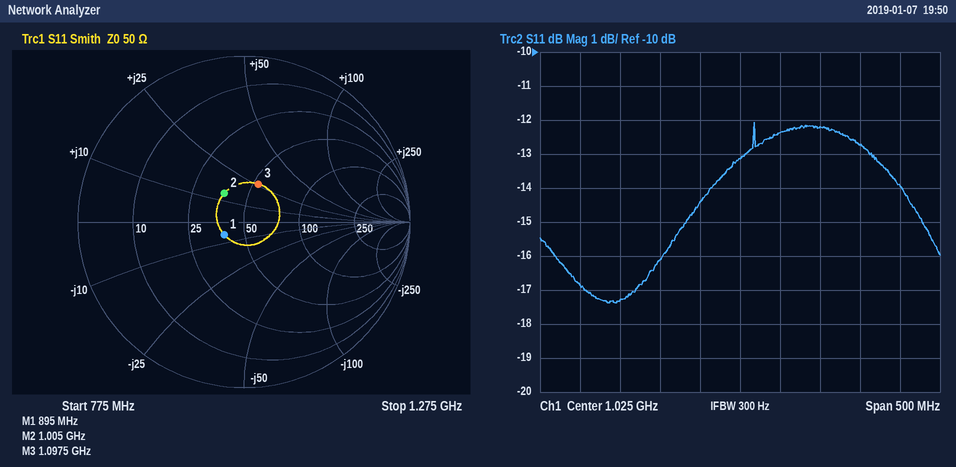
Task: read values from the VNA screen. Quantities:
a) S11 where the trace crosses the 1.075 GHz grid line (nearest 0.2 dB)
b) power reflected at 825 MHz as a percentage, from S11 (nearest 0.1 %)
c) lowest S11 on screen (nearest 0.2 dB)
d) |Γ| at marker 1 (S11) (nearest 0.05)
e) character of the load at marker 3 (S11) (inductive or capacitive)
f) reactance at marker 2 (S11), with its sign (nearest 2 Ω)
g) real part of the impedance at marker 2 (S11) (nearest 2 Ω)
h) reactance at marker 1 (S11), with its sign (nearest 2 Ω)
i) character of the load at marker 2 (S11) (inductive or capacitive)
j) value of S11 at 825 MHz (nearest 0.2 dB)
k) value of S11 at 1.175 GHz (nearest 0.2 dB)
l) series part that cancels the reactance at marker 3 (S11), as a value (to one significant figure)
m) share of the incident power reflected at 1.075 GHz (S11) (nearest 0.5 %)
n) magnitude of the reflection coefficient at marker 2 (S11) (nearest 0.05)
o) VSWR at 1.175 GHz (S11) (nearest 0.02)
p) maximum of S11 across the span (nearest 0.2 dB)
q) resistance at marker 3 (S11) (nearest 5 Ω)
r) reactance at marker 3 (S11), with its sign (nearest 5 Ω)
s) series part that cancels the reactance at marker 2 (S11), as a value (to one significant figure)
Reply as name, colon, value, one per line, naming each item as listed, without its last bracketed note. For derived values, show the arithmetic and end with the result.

S11 where the trace crosses the 1.075 GHz grid line: -12.4 dB
power reflected at 825 MHz as a percentage, from S11: 10^(-16.8/10) ≈ 2.1 %
lowest S11 on screen: -17.4 dB
|Γ| at marker 1 (S11): 0.15
character of the load at marker 3 (S11): inductive
reactance at marker 2 (S11), with its sign: +14 Ω
real part of the impedance at marker 2 (S11): 38 Ω
reactance at marker 1 (S11), with its sign: -6 Ω
character of the load at marker 2 (S11): inductive
value of S11 at 825 MHz: -16.8 dB
value of S11 at 1.175 GHz: -12.8 dB
series part that cancels the reactance at marker 3 (S11), as a value: C = 1/(2π × 1.0975 GHz × 25 Ω) ≈ 6 pF
share of the incident power reflected at 1.075 GHz (S11): 10^(-12.4/10) ≈ 5.75 %, so 6.0 % to the nearest 0.5 %
magnitude of the reflection coefficient at marker 2 (S11): 0.20
VSWR at 1.175 GHz (S11): |Γ| = 10^(-12.8/20) = 0.2291; VSWR = (1 + 0.2291)/(1 − 0.2291) ≈ 1.59, so 1.60 to the nearest 0.02
maximum of S11 across the span: -12.0 dB
resistance at marker 3 (S11): 55 Ω
reactance at marker 3 (S11), with its sign: +25 Ω
series part that cancels the reactance at marker 2 (S11), as a value: C = 1/(2π × 1.005 GHz × 14 Ω) ≈ 11.3 pF, so 10 pF to one significant figure
